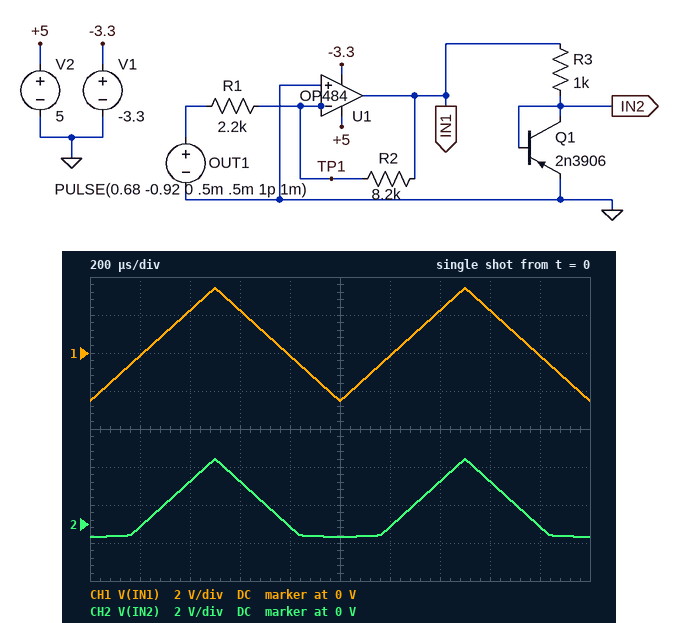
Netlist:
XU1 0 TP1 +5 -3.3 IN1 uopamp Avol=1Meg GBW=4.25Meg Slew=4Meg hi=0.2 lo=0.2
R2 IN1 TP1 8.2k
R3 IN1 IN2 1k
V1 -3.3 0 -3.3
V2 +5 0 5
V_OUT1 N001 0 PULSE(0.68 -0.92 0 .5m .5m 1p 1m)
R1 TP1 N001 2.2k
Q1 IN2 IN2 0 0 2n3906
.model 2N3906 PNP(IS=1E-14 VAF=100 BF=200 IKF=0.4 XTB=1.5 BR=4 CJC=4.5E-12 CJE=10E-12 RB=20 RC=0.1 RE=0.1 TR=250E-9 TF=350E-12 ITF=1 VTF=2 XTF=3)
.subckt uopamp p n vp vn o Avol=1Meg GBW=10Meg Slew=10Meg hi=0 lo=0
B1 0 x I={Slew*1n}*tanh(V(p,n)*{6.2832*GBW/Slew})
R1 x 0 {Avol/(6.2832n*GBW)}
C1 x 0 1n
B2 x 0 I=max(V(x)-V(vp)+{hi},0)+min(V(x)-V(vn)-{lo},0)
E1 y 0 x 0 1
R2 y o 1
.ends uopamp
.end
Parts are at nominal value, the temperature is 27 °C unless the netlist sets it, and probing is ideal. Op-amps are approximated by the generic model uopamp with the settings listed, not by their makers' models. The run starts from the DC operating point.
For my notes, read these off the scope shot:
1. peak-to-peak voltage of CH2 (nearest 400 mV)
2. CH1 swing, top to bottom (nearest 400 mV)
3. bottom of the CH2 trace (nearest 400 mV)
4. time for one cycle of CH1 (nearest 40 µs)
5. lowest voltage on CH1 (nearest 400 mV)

4.0 V
6.0 V
-800 mV
1.00 ms
-2.4 V
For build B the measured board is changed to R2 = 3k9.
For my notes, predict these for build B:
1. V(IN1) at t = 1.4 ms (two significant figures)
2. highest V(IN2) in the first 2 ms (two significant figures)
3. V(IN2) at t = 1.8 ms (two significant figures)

1.1 V
1.6 V
-70 mV
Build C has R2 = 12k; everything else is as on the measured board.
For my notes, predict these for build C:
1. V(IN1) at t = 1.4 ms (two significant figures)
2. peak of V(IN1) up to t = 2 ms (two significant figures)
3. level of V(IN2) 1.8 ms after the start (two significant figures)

3.3 V
4.8 V
-210 mV
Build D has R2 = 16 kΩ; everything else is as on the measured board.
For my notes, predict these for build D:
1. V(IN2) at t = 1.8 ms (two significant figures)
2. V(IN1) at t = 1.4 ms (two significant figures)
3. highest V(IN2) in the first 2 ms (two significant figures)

-280 mV
4.4 V
4.8 V
